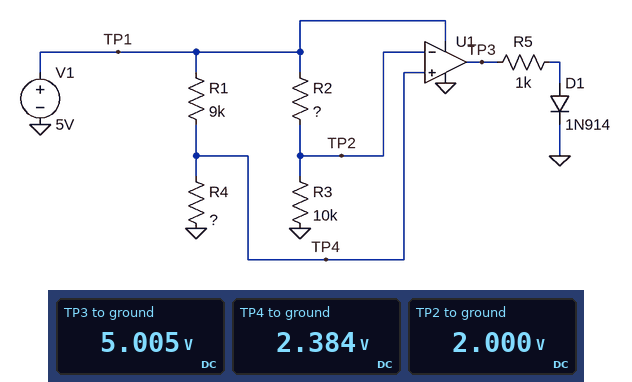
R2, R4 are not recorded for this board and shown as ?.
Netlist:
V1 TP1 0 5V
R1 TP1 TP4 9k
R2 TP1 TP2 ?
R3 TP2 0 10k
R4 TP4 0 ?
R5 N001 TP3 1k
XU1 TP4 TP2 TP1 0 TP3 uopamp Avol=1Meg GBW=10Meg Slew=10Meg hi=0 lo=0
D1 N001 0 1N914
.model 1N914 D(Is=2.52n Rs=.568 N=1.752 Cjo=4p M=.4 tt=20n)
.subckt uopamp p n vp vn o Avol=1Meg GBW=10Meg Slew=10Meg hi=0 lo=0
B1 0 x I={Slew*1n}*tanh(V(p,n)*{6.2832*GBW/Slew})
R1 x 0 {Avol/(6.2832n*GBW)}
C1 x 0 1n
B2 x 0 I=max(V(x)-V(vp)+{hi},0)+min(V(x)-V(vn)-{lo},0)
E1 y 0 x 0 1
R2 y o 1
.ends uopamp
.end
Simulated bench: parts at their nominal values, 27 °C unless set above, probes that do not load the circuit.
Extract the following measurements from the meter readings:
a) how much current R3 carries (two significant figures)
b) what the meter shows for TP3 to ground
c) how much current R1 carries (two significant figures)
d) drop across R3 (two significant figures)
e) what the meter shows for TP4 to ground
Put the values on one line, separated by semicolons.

200 µA; 5.005 V; 290 µA; 2.0 V; 2.384 V
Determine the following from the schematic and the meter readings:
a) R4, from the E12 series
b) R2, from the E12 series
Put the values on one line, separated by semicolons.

8.2 kΩ; 15 kΩ
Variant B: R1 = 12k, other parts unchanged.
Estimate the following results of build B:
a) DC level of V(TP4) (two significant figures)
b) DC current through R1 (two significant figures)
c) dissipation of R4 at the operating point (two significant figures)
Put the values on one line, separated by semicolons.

2.0 V; 250 µA; 500 µW
